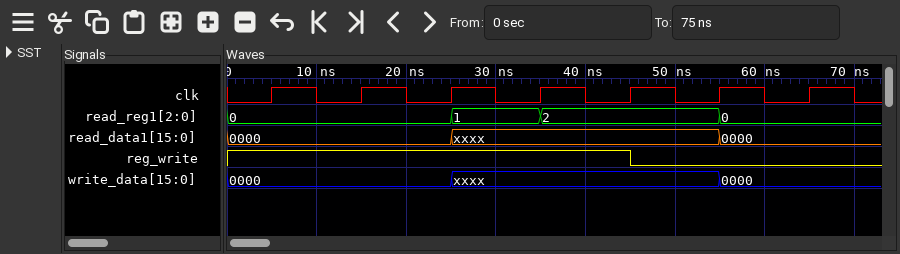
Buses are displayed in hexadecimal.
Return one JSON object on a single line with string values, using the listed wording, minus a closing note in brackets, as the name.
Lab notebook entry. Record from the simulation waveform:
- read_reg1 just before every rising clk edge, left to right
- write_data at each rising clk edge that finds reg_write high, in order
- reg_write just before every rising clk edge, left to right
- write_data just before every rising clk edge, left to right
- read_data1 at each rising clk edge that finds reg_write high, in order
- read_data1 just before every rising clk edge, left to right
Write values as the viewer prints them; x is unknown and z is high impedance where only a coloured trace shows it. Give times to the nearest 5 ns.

{"read_reg1 just before every rising clk edge, left to right": "0, 0, 0, 1, 2, 2, 0", "write_data at each rising clk edge that finds reg_write high, in order": "0000, 0000, 0000, xxxx, xxxx", "reg_write just before every rising clk edge, left to right": "1 1 1 1 1 0 0", "write_data just before every rising clk edge, left to right": "0000, 0000, 0000, xxxx, xxxx, xxxx, 0000", "read_data1 at each rising clk edge that finds reg_write high, in order": "0000, 0000, 0000, xxxx, xxxx", "read_data1 just before every rising clk edge, left to right": "0000, 0000, 0000, xxxx, xxxx, xxxx, 0000"}
